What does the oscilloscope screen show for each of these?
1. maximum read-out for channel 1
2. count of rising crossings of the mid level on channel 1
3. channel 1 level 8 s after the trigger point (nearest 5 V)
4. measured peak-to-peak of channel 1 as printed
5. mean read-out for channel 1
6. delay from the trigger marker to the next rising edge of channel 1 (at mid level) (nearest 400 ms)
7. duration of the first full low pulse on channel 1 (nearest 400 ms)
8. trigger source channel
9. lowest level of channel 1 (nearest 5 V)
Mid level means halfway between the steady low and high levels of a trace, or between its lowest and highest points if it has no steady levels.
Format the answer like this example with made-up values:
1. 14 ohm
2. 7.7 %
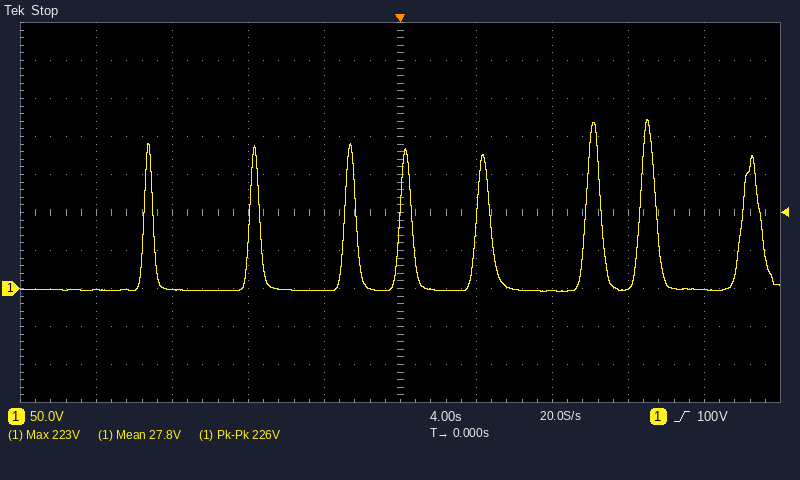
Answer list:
1. 223 V
2. 8
3. -5 V
4. 226 V
5. 27.8 V
6. 4.0 s
7. 5.2 s
8. channel 1
9. -5 V
